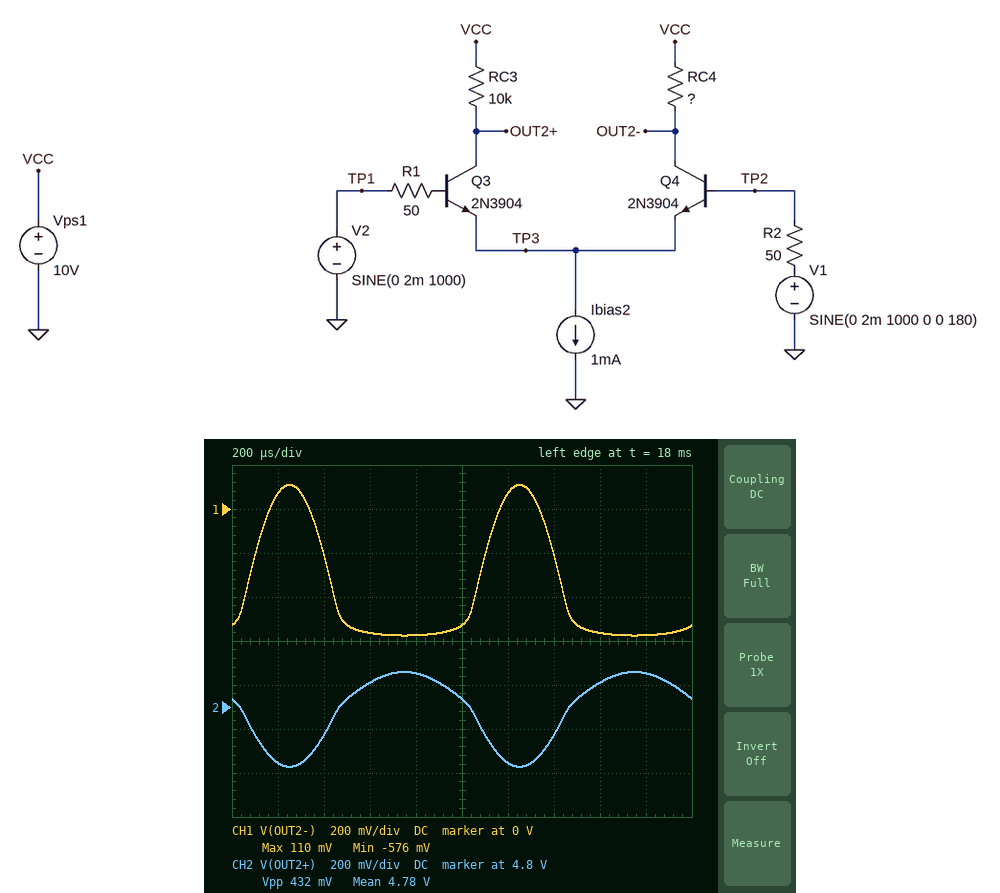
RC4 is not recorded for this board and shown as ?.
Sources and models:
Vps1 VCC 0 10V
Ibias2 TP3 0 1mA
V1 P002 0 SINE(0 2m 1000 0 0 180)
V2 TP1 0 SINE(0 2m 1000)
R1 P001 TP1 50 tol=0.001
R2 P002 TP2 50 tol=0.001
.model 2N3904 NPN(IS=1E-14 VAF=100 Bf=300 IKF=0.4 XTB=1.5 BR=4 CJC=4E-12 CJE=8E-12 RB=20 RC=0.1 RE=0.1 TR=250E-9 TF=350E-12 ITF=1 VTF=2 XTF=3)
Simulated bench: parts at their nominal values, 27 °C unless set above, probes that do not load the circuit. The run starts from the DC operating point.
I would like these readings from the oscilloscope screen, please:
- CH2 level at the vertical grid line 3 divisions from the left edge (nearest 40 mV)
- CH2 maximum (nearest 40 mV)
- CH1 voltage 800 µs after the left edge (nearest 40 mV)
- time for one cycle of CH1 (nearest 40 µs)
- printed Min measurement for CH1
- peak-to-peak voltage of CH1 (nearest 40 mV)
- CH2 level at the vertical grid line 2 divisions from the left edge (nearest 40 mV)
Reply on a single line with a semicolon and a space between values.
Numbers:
4.92 V; 4.96 V; -560 mV; 1.00 ms; -576 mV; 680 mV; 4.68 V
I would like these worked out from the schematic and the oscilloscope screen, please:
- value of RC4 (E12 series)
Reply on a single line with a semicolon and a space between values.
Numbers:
22 kΩ
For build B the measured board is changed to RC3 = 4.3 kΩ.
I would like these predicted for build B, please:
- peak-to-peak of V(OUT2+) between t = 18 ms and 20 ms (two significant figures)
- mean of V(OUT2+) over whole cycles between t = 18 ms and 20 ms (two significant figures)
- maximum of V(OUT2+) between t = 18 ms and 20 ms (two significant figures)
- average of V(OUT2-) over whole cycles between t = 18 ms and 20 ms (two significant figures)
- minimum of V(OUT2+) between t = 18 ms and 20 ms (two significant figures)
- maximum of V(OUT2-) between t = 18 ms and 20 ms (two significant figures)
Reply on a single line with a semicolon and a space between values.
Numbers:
210 mV; 7.7 V; 7.8 V; -290 mV; 7.6 V; 260 mV
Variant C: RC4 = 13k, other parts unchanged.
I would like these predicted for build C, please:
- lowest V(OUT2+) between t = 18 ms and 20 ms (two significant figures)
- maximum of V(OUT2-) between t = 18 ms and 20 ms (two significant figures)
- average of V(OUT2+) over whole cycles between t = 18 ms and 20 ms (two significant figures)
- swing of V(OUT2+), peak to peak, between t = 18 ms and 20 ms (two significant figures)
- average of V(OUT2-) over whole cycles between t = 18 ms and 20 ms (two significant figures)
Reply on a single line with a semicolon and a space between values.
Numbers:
4.6 V; 4.0 V; 5.0 V; 720 mV; 3.6 V
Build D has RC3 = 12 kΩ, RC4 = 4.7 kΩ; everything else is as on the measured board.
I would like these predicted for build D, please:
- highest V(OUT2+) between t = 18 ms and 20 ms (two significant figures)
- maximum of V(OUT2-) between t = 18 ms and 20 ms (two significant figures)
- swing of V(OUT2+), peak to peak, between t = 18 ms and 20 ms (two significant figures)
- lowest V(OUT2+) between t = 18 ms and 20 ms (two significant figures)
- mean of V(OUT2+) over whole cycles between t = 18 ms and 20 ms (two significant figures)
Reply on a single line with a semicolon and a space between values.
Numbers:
4.6 V; 7.8 V; 880 mV; 3.7 V; 4.1 V
